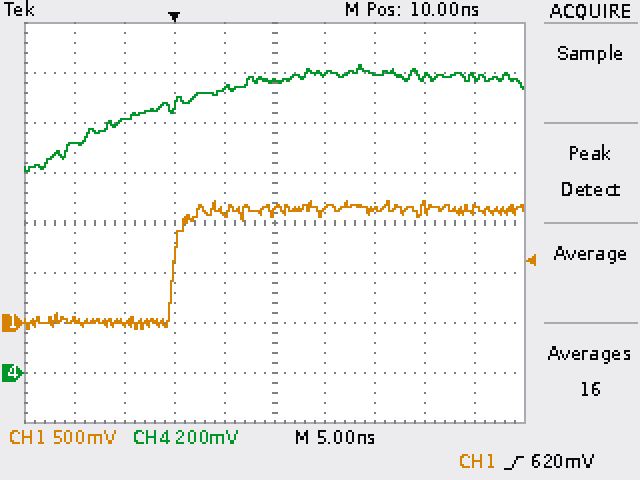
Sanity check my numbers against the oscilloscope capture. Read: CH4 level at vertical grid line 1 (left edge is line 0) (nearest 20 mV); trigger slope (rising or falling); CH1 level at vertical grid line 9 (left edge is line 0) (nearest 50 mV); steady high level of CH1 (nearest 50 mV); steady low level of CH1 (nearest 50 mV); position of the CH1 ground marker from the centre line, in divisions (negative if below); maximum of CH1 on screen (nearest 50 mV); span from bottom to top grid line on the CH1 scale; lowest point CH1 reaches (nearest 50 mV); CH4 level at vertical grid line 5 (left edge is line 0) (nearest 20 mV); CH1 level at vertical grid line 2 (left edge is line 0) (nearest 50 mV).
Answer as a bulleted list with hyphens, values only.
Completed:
- 920 mV
- rising
- 1.15 V
- 1.15 V
- 0 mV
- -2.0 div
- 1.20 V
- 4 V
- -50 mV
- 1.16 V
- 0 mV
